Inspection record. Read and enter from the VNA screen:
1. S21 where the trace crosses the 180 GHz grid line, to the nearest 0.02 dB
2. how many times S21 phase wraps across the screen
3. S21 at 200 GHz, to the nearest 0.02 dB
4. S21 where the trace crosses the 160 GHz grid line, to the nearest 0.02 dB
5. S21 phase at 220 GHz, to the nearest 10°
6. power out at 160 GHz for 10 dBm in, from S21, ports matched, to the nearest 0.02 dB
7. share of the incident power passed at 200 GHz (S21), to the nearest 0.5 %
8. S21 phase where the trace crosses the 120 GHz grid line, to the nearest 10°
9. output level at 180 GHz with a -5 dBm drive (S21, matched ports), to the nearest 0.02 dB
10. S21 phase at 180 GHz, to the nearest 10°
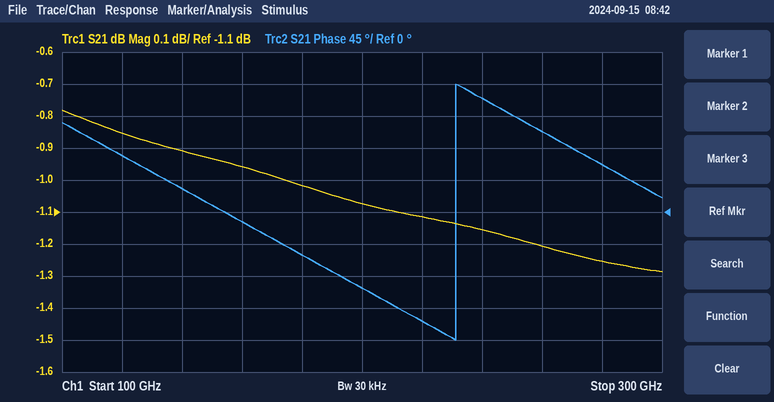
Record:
-1.02 dB
1
-1.08 dB
-0.96 dB
-150°
9.04 dBm
78.0 %
80°
-6.02 dBm
-60°
